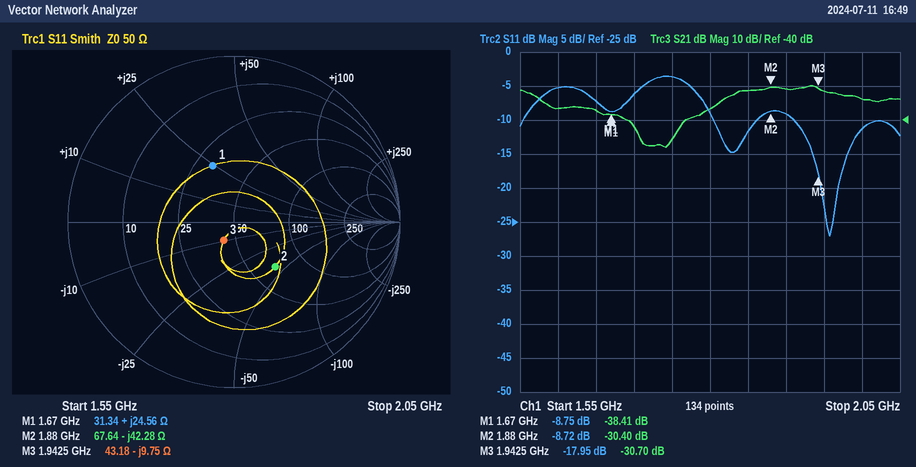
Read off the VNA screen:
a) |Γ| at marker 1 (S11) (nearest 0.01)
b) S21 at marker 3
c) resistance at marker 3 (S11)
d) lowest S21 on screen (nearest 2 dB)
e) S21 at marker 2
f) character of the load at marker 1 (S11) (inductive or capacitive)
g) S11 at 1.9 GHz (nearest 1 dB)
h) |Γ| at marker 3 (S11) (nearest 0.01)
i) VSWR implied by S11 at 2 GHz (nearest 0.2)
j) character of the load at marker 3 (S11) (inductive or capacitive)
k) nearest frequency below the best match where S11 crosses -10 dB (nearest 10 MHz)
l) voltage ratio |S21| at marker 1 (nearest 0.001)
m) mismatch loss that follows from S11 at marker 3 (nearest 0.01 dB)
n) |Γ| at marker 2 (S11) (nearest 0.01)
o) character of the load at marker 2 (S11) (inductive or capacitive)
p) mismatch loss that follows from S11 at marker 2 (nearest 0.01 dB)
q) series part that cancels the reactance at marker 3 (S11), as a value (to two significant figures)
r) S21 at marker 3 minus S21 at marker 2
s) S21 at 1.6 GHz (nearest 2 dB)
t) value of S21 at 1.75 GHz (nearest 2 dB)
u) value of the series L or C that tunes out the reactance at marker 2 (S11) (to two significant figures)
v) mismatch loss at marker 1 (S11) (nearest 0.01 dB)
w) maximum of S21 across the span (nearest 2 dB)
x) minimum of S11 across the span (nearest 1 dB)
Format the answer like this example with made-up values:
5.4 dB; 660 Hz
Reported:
0.36; -30.70 dB; 43.18 Ω; -48 dB; -30.40 dB; inductive; -9 dB; 0.13; 1.8; capacitive; 1.91 GHz; 0.012; 0.07 dB; 0.37; capacitive; 0.63 dB; 800 pH; -0.30 dB; -36 dB; -46 dB; 3.6 nH; 0.62 dB; -30 dB; -27 dB
